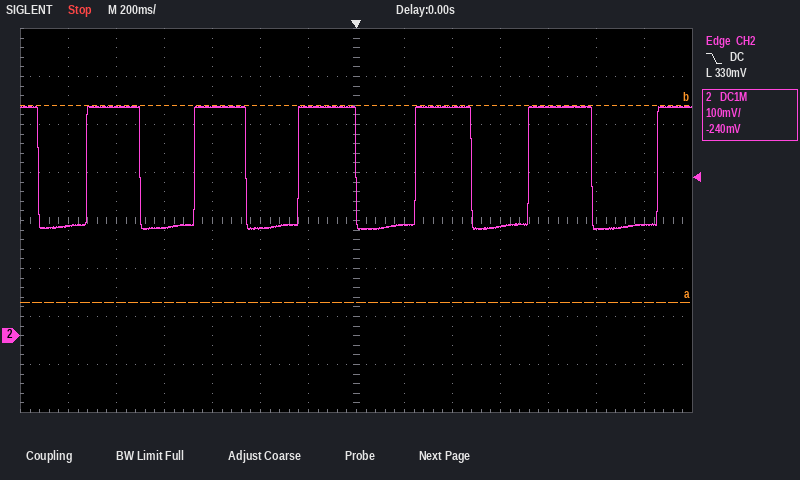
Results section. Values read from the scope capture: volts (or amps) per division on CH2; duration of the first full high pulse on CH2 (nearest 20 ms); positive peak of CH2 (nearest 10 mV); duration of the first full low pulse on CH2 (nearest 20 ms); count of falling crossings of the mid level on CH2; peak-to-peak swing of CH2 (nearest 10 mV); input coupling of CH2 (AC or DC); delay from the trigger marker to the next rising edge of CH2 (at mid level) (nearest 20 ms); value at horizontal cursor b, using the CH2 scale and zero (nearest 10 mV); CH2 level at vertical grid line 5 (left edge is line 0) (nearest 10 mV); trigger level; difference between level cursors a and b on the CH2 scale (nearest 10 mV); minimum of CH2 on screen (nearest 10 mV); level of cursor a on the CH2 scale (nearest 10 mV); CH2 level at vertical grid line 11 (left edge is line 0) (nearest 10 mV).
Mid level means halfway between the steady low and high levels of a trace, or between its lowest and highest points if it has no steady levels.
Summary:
100 mV
220 ms
480 mV
200 ms
6
260 mV
DC
240 ms
480 mV
220 mV
330 mV
410 mV
220 mV
70 mV
480 mV
